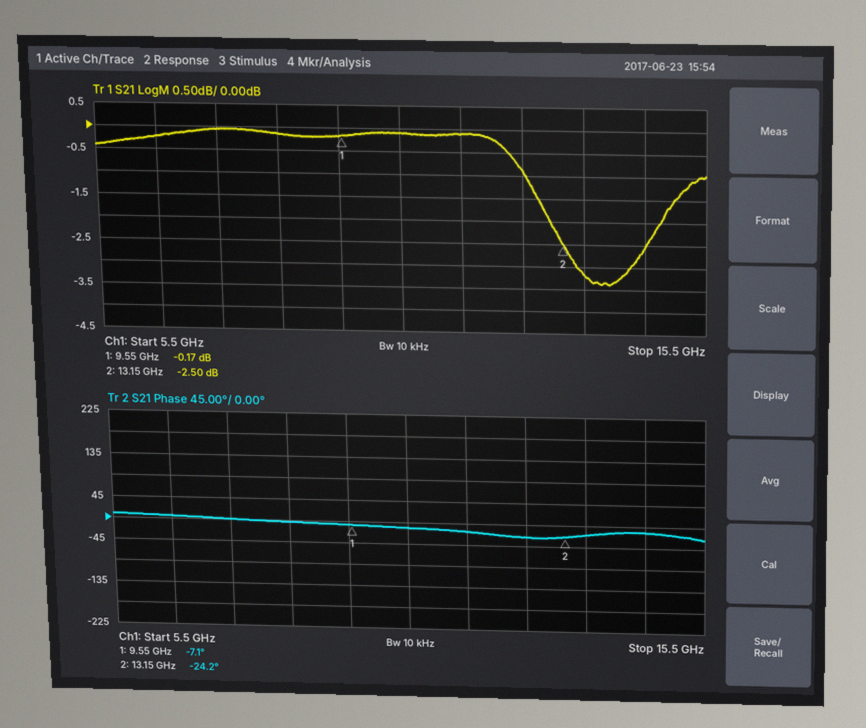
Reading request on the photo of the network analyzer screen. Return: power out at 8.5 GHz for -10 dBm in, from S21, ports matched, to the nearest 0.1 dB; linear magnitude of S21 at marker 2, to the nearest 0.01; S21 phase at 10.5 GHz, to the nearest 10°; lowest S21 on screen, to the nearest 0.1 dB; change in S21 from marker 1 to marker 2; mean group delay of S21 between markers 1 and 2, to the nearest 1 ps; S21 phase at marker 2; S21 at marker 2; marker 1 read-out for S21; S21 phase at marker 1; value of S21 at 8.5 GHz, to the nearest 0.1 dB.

-10.1 dBm
0.75
-10°
-3.4 dB
-2.33 dB
13 ps
-24.2°
-2.50 dB
-0.17 dB
-7.1°
-0.1 dB
